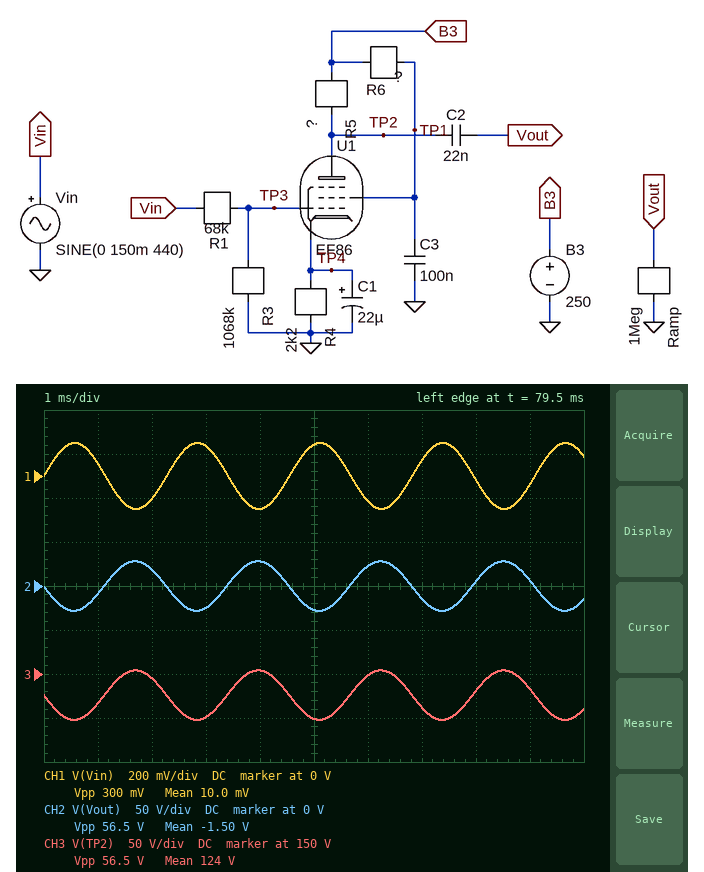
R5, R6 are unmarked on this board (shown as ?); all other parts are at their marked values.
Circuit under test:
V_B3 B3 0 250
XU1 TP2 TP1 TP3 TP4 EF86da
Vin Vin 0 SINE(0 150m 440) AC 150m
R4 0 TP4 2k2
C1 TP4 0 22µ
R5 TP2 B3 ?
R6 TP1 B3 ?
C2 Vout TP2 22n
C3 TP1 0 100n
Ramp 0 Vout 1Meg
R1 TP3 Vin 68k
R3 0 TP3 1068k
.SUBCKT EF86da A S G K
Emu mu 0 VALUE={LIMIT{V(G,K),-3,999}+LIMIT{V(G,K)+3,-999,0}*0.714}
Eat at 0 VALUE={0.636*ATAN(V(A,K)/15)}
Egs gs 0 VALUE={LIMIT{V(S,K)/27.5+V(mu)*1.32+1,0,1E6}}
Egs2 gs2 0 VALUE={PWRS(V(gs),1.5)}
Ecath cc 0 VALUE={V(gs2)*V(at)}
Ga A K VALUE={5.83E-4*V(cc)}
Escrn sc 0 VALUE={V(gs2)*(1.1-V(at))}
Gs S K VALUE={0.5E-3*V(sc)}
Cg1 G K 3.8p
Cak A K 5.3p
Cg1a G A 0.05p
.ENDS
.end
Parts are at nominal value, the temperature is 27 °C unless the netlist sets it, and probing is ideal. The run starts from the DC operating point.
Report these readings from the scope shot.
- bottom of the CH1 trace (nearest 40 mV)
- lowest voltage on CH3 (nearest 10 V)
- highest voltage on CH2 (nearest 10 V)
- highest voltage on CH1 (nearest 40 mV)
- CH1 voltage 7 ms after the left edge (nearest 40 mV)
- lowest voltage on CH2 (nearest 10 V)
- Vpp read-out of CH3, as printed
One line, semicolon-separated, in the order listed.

-160 mV; 100 V; 30 V; 160 mV; 80 mV; -30 V; 56.5 V
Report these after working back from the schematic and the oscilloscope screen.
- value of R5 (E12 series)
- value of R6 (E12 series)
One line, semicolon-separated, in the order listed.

270 kΩ; 2.7 MΩ
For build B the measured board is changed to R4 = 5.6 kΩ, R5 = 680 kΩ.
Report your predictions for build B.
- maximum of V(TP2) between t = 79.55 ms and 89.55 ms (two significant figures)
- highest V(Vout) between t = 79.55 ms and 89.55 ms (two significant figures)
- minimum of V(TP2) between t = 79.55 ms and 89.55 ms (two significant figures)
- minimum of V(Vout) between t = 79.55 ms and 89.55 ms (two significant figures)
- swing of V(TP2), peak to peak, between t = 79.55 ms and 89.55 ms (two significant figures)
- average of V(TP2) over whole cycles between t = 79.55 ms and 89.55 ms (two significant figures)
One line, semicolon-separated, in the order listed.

110 V; 37 V; 40 V; -32 V; 70 V; 73 V
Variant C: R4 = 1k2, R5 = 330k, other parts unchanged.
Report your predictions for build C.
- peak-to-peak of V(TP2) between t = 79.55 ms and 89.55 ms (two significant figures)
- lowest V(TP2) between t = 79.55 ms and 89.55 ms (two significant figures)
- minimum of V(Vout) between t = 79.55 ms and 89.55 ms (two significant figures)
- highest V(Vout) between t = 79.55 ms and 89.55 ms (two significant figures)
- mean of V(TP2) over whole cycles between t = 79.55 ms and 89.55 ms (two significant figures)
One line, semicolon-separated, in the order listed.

61 V; 73 V; -30 V; 31 V; 100 V
